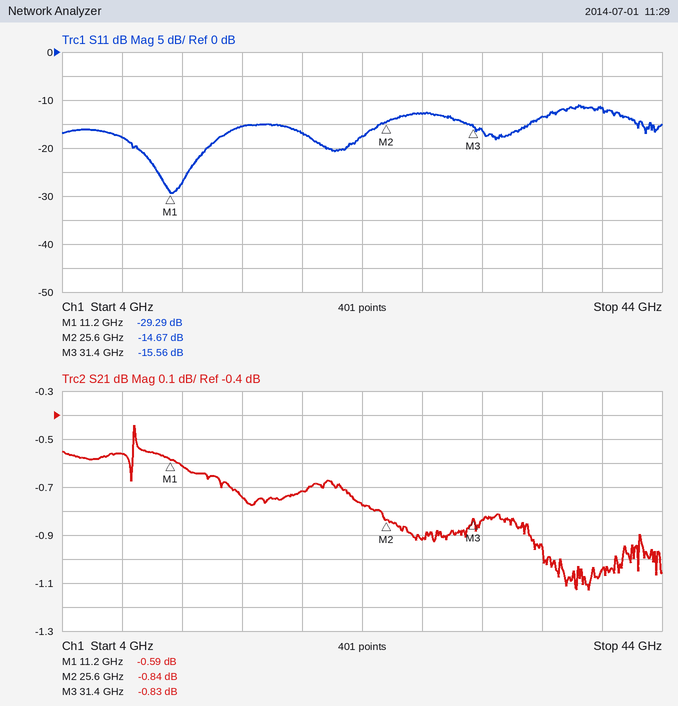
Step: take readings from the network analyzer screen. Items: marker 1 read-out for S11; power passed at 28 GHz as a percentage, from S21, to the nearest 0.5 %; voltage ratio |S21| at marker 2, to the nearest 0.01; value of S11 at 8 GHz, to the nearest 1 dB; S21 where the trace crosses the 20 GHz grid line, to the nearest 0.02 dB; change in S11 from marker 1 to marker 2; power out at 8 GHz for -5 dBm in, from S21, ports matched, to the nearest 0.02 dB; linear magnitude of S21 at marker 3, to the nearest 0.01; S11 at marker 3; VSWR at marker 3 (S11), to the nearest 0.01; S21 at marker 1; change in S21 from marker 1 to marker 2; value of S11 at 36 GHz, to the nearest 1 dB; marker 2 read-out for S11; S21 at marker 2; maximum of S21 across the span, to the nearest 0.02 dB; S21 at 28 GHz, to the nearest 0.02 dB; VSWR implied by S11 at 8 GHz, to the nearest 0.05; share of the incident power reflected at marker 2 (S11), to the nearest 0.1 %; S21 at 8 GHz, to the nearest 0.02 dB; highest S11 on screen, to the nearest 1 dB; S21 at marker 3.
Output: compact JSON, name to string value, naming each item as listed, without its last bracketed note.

{"marker 1 read-out for S11": "-29.29 dB", "power passed at 28 GHz as a percentage, from S21, to the nearest 0.5 %": "81.0 %", "voltage ratio |S21| at marker 2, to the nearest 0.01": "0.91", "value of S11 at 8 GHz, to the nearest 1 dB": "-18 dB", "S21 where the trace crosses the 20 GHz grid line, to the nearest 0.02 dB": "-0.72 dB", "change in S11 from marker 1 to marker 2": "14.62 dB", "power out at 8 GHz for -5 dBm in, from S21, ports matched, to the nearest 0.02 dB": "-5.56 dBm", "linear magnitude of S21 at marker 3, to the nearest 0.01": "0.91", "S11 at marker 3": "-15.56 dB", "VSWR at marker 3 (S11), to the nearest 0.01": "1.40", "S21 at marker 1": "-0.59 dB", "change in S21 from marker 1 to marker 2": "-0.25 dB", "value of S11 at 36 GHz, to the nearest 1 dB": "-13 dB", "marker 2 read-out for S11": "-14.67 dB", "S21 at marker 2": "-0.84 dB", "maximum of S21 across the span, to the nearest 0.02 dB": "-0.44 dB", "S21 at 28 GHz, to the nearest 0.02 dB": "-0.92 dB", "VSWR implied by S11 at 8 GHz, to the nearest 0.05": "1.30", "share of the incident power reflected at marker 2 (S11), to the nearest 0.1 %": "3.4 %", "S21 at 8 GHz, to the nearest 0.02 dB": "-0.56 dB", "highest S11 on screen, to the nearest 1 dB": "-11 dB", "S21 at marker 3": "-0.83 dB"}
